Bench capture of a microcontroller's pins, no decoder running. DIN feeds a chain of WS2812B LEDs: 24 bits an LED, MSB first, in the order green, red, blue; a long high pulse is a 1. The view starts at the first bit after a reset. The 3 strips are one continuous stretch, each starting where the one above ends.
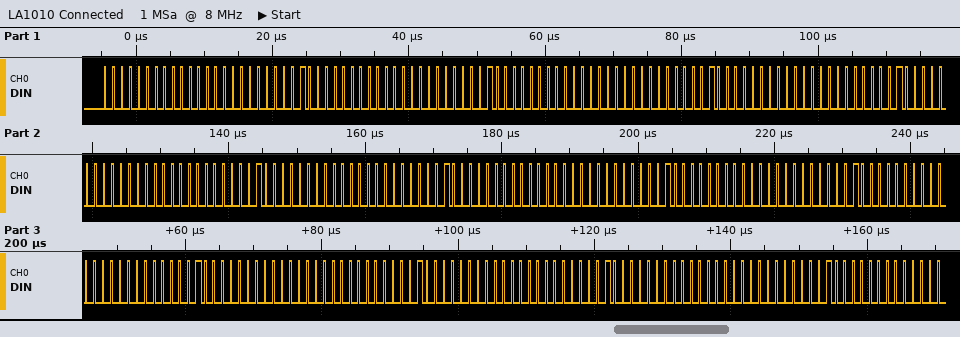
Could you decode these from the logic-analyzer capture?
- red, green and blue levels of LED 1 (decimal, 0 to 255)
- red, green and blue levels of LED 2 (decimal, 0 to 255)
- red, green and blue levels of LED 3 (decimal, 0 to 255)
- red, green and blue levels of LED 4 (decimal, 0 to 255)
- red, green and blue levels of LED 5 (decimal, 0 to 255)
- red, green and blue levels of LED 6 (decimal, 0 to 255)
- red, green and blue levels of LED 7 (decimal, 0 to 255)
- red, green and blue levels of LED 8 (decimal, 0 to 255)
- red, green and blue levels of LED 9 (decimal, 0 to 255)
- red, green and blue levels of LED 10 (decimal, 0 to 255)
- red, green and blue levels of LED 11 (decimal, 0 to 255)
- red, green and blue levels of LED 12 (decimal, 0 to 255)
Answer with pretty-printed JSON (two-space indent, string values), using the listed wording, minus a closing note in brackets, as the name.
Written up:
{
  "red, green and blue levels of LED 1": "0, 0, 1",
  "red, green and blue levels of LED 2": "0, 0, 4",
  "red, green and blue levels of LED 3": "0, 0, 1",
  "red, green and blue levels of LED 4": "0, 0, 4",
  "red, green and blue levels of LED 5": "0, 0, 1",
  "red, green and blue levels of LED 6": "0, 0, 4",
  "red, green and blue levels of LED 7": "0, 0, 1",
  "red, green and blue levels of LED 8": "0, 0, 4",
  "red, green and blue levels of LED 9": "0, 0, 4",
  "red, green and blue levels of LED 10": "0, 0, 1",
  "red, green and blue levels of LED 11": "0, 0, 4",
  "red, green and blue levels of LED 12": "0, 0, 1"
}
